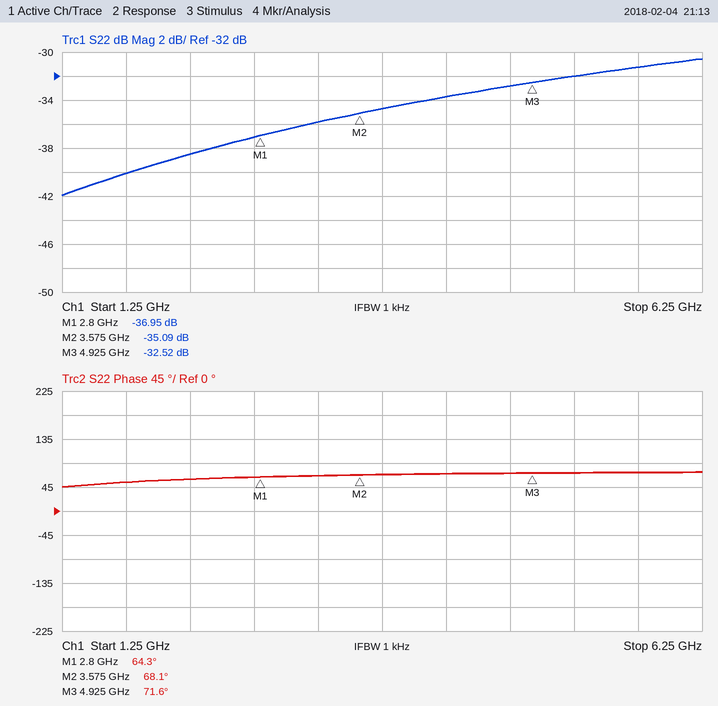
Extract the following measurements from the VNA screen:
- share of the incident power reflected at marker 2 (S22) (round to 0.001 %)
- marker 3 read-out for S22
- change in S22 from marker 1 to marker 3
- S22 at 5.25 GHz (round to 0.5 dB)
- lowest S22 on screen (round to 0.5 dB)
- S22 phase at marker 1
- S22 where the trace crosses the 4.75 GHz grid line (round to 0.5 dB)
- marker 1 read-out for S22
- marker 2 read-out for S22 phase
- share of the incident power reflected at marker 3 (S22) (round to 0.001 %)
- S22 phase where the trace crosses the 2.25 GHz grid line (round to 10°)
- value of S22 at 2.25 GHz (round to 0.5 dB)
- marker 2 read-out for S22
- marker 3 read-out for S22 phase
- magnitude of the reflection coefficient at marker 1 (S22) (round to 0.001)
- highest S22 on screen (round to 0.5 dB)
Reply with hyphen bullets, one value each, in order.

- 0.031 %
- -32.52 dB
- 4.43 dB
- -32.0 dB
- -42.0 dB
- 64.3°
- -33.0 dB
- -36.95 dB
- 68.1°
- 0.056 %
- 60°
- -38.5 dB
- -35.09 dB
- 71.6°
- 0.014
- -30.5 dB
